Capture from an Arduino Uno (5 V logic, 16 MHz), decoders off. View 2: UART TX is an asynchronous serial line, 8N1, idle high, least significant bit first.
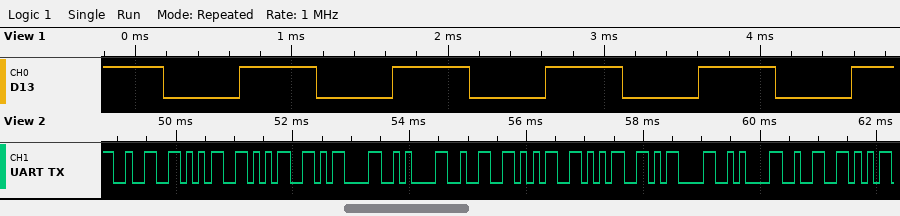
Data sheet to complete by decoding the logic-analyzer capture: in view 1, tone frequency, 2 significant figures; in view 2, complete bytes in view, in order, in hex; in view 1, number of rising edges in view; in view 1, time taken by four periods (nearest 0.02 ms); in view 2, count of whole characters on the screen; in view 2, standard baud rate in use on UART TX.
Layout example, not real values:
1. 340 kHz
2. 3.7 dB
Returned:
1. 1.0 kHz
2. 32 35 35 0D 0A 32 35 35 0D 0A 32
3. 5
4. 3.92 ms
5. 11
6. 9600 baud
